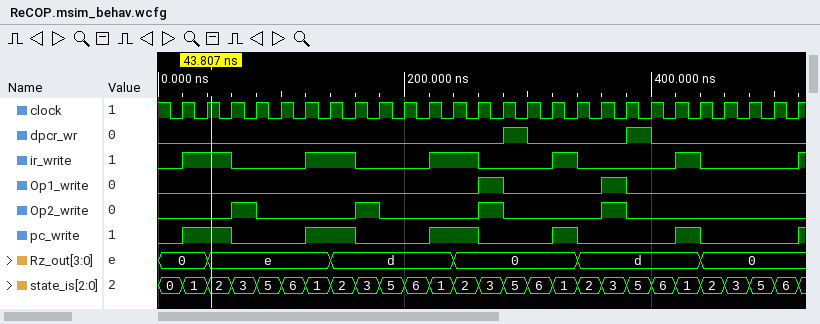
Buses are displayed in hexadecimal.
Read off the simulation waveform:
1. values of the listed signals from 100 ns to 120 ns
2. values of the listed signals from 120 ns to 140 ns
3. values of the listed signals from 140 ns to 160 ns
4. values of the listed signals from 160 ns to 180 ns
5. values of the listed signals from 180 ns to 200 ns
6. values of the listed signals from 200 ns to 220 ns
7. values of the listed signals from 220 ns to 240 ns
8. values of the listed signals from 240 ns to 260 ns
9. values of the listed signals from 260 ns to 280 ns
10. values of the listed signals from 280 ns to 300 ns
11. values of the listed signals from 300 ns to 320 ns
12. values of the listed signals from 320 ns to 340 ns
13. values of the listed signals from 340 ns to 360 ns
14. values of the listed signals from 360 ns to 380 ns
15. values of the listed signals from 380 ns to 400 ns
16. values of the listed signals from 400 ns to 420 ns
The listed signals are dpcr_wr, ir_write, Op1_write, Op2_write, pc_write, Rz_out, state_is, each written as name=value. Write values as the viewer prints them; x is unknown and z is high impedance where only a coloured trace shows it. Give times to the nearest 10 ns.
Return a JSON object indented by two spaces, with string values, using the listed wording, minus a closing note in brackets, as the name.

{
  "values of the listed signals from 100 ns to 120 ns": "dpcr_wr=0, ir_write=0, Op1_write=0, Op2_write=0, pc_write=0, Rz_out=e, state_is=6",
  "values of the listed signals from 120 ns to 140 ns": "dpcr_wr=0, ir_write=1, Op1_write=0, Op2_write=0, pc_write=1, Rz_out=e, state_is=1",
  "values of the listed signals from 140 ns to 160 ns": "dpcr_wr=0, ir_write=1, Op1_write=0, Op2_write=0, pc_write=1, Rz_out=d, state_is=2",
  "values of the listed signals from 160 ns to 180 ns": "dpcr_wr=0, ir_write=0, Op1_write=0, Op2_write=1, pc_write=0, Rz_out=d, state_is=3",
  "values of the listed signals from 180 ns to 200 ns": "dpcr_wr=0, ir_write=0, Op1_write=0, Op2_write=0, pc_write=0, Rz_out=d, state_is=5",
  "values of the listed signals from 200 ns to 220 ns": "dpcr_wr=0, ir_write=0, Op1_write=0, Op2_write=0, pc_write=0, Rz_out=d, state_is=6",
  "values of the listed signals from 220 ns to 240 ns": "dpcr_wr=0, ir_write=1, Op1_write=0, Op2_write=0, pc_write=1, Rz_out=d, state_is=1",
  "values of the listed signals from 240 ns to 260 ns": "dpcr_wr=0, ir_write=1, Op1_write=0, Op2_write=0, pc_write=1, Rz_out=0, state_is=2",
  "values of the listed signals from 260 ns to 280 ns": "dpcr_wr=0, ir_write=0, Op1_write=1, Op2_write=1, pc_write=0, Rz_out=0, state_is=3",
  "values of the listed signals from 280 ns to 300 ns": "dpcr_wr=1, ir_write=0, Op1_write=0, Op2_write=0, pc_write=0, Rz_out=0, state_is=5",
  "values of the listed signals from 300 ns to 320 ns": "dpcr_wr=0, ir_write=0, Op1_write=0, Op2_write=0, pc_write=0, Rz_out=0, state_is=6",
  "values of the listed signals from 320 ns to 340 ns": "dpcr_wr=0, ir_write=1, Op1_write=0, Op2_write=0, pc_write=1, Rz_out=0, state_is=1",
  "values of the listed signals from 340 ns to 360 ns": "dpcr_wr=0, ir_write=0, Op1_write=0, Op2_write=0, pc_write=0, Rz_out=d, state_is=2",
  "values of the listed signals from 360 ns to 380 ns": "dpcr_wr=0, ir_write=0, Op1_write=1, Op2_write=1, pc_write=0, Rz_out=d, state_is=3",
  "values of the listed signals from 380 ns to 400 ns": "dpcr_wr=1, ir_write=0, Op1_write=0, Op2_write=0, pc_write=0, Rz_out=d, state_is=5",
  "values of the listed signals from 400 ns to 420 ns": "dpcr_wr=0, ir_write=0, Op1_write=0, Op2_write=0, pc_write=0, Rz_out=d, state_is=6"
}
